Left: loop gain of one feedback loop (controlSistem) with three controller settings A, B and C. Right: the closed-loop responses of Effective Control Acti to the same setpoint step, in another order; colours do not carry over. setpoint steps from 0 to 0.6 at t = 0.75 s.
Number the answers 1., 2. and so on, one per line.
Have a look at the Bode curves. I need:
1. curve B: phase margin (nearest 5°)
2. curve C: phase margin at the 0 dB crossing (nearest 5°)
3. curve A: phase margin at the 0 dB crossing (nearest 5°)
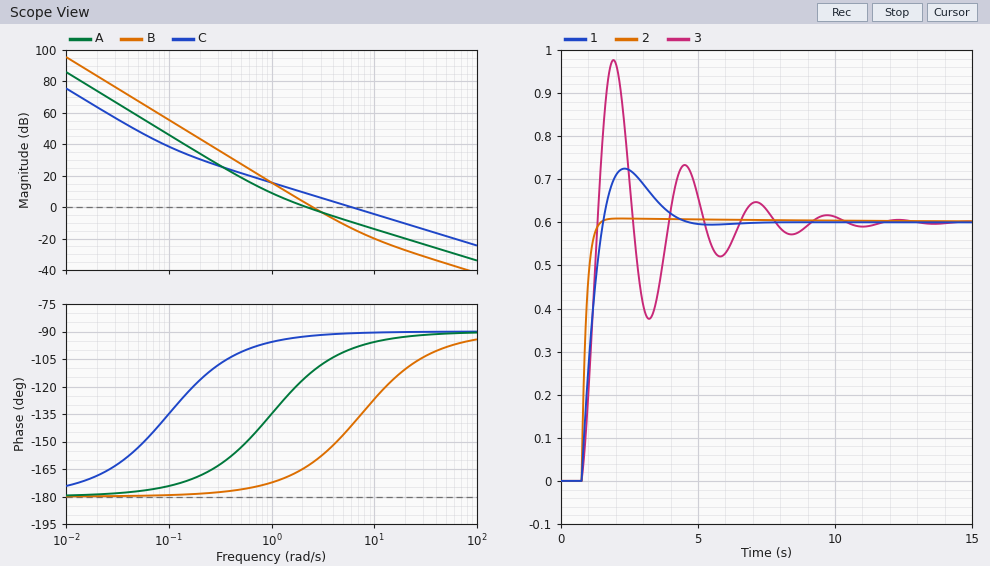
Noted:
1. 20°
2. 90°
3. 65°
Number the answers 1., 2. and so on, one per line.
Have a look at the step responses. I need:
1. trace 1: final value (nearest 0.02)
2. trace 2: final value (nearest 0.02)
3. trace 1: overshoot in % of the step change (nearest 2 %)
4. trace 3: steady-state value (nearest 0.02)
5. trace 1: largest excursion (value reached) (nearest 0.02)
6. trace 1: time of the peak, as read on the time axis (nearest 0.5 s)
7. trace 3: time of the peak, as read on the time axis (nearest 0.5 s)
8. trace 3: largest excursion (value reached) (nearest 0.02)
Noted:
1. 0.60
2. 0.60
3. 20 %
4. 0.60
5. 0.72
6. 2.5 s
7. 2.0 s
8. 0.98
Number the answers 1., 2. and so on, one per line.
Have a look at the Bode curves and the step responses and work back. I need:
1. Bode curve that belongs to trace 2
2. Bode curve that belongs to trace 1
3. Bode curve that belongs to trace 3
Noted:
1. C
2. A
3. B
